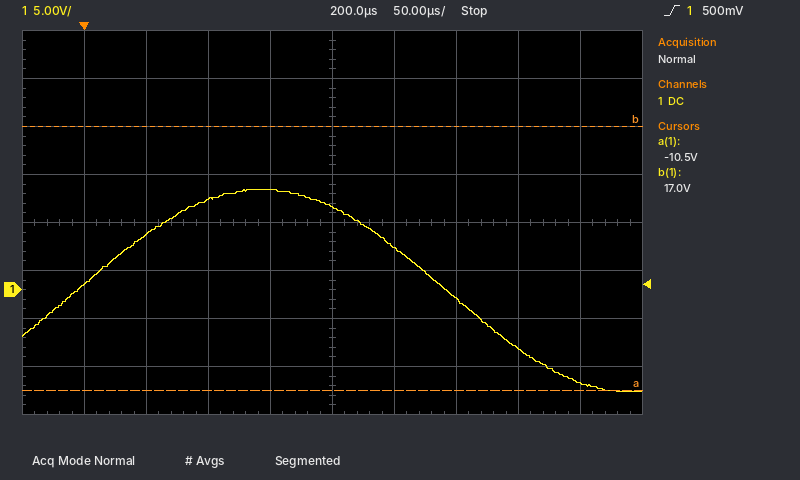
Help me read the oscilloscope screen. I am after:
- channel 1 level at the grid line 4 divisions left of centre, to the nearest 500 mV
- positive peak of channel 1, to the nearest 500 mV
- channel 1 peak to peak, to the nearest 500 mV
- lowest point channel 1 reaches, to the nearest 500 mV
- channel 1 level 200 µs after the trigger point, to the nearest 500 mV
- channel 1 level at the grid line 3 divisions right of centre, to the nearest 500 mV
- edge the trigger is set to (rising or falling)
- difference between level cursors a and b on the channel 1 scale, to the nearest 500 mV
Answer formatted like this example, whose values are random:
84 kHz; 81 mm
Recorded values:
500 mV; 10.5 V; 21.0 V; -10.5 V; 8.5 V; -6.0 V; rising; 27.5 V
